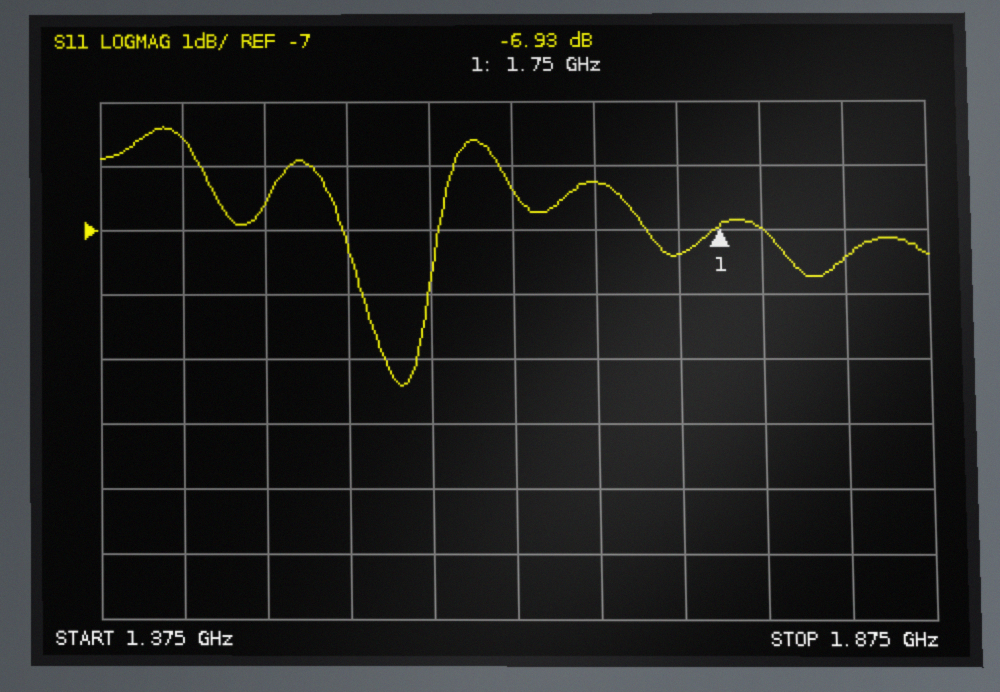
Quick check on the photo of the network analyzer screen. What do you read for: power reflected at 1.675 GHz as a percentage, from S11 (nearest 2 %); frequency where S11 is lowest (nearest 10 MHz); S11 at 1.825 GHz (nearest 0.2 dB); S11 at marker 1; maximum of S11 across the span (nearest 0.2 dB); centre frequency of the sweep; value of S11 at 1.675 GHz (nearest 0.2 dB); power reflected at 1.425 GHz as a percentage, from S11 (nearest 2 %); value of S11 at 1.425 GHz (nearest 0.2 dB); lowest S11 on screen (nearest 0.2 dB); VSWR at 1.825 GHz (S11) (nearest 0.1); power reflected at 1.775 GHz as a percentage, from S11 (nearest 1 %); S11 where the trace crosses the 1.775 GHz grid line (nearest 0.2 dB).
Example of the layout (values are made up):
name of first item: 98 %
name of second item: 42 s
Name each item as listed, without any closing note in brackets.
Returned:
power reflected at 1.675 GHz as a percentage, from S11: 24 %
frequency where S11 is lowest: 1.56 GHz
S11 at 1.825 GHz: -7.4 dB
S11 at marker 1: -6.93 dB
maximum of S11 across the span: -5.4 dB
centre frequency of the sweep: 1.625 GHz
value of S11 at 1.675 GHz: -6.2 dB
power reflected at 1.425 GHz as a percentage, from S11: 28 %
value of S11 at 1.425 GHz: -5.6 dB
lowest S11 on screen: -9.4 dB
VSWR at 1.825 GHz (S11): 2.5
power reflected at 1.775 GHz as a percentage, from S11: 20 %
S11 where the trace crosses the 1.775 GHz grid line: -7.0 dB
